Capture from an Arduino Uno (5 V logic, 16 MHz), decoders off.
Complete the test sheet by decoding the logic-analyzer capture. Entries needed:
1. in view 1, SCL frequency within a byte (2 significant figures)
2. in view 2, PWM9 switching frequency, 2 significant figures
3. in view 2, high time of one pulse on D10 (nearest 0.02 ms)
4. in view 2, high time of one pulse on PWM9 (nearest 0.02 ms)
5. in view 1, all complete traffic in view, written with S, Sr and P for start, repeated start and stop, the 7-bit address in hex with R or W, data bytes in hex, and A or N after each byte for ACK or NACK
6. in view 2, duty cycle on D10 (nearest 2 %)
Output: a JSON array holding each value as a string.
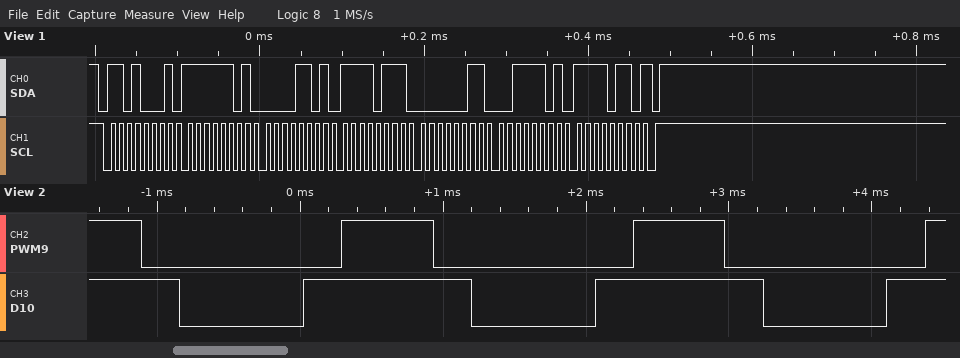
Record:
["100 kHz", "490 Hz", "1.18 ms", "0.64 ms", "S 68R A FD A 0D A F7 A 03 A 3D A F6 N P", "58 %"]
